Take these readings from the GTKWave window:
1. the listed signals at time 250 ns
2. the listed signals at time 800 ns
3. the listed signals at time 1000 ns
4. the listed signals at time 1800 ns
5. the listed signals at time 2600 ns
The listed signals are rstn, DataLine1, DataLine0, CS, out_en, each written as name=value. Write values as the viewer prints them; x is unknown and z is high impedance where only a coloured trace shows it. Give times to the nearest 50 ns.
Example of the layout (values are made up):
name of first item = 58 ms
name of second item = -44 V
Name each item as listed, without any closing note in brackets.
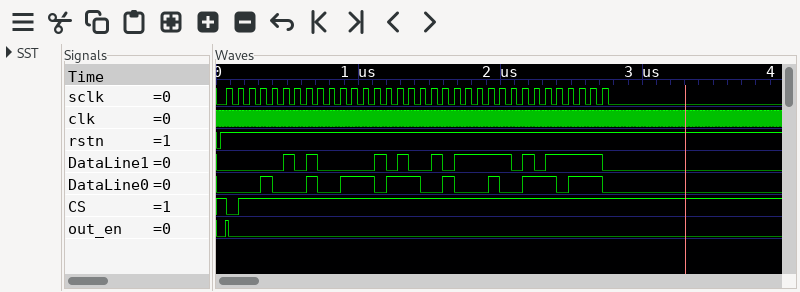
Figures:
the listed signals at time 250 ns = rstn=1, DataLine1=0, DataLine0=0, CS=1, out_en=0
the listed signals at time 800 ns = rstn=1, DataLine1=0, DataLine0=0, CS=1, out_en=0
the listed signals at time 1000 ns = rstn=1, DataLine1=0, DataLine0=1, CS=1, out_en=0
the listed signals at time 1800 ns = rstn=1, DataLine1=1, DataLine0=0, CS=1, out_en=0
the listed signals at time 2600 ns = rstn=1, DataLine1=1, DataLine0=1, CS=1, out_en=0
